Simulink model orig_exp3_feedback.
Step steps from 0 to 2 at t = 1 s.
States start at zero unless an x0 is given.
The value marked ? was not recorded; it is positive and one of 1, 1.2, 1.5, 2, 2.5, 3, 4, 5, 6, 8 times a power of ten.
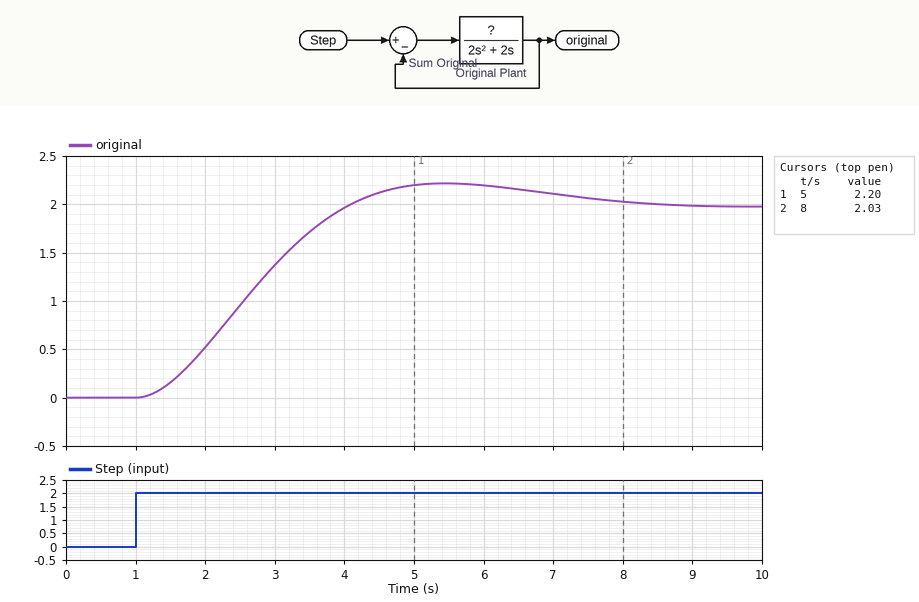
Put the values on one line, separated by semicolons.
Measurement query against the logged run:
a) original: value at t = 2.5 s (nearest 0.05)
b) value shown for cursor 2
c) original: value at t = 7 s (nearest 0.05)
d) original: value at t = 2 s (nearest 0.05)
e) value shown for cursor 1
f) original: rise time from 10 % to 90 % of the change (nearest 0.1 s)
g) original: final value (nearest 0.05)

0.95; 2.03; 2.10; 0.50; 2.20; 2.1 s; 2.00
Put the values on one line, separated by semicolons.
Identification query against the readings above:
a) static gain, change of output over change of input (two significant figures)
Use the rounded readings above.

1.0
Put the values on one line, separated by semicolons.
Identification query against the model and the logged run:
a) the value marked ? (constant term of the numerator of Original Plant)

1.5
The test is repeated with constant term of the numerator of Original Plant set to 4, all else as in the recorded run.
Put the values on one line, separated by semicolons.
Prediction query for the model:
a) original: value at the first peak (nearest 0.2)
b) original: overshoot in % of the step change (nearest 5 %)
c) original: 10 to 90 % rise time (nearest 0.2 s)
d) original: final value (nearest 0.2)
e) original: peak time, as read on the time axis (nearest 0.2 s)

2.6; 30 %; 1.0 s; 2.0; 3.4 s
